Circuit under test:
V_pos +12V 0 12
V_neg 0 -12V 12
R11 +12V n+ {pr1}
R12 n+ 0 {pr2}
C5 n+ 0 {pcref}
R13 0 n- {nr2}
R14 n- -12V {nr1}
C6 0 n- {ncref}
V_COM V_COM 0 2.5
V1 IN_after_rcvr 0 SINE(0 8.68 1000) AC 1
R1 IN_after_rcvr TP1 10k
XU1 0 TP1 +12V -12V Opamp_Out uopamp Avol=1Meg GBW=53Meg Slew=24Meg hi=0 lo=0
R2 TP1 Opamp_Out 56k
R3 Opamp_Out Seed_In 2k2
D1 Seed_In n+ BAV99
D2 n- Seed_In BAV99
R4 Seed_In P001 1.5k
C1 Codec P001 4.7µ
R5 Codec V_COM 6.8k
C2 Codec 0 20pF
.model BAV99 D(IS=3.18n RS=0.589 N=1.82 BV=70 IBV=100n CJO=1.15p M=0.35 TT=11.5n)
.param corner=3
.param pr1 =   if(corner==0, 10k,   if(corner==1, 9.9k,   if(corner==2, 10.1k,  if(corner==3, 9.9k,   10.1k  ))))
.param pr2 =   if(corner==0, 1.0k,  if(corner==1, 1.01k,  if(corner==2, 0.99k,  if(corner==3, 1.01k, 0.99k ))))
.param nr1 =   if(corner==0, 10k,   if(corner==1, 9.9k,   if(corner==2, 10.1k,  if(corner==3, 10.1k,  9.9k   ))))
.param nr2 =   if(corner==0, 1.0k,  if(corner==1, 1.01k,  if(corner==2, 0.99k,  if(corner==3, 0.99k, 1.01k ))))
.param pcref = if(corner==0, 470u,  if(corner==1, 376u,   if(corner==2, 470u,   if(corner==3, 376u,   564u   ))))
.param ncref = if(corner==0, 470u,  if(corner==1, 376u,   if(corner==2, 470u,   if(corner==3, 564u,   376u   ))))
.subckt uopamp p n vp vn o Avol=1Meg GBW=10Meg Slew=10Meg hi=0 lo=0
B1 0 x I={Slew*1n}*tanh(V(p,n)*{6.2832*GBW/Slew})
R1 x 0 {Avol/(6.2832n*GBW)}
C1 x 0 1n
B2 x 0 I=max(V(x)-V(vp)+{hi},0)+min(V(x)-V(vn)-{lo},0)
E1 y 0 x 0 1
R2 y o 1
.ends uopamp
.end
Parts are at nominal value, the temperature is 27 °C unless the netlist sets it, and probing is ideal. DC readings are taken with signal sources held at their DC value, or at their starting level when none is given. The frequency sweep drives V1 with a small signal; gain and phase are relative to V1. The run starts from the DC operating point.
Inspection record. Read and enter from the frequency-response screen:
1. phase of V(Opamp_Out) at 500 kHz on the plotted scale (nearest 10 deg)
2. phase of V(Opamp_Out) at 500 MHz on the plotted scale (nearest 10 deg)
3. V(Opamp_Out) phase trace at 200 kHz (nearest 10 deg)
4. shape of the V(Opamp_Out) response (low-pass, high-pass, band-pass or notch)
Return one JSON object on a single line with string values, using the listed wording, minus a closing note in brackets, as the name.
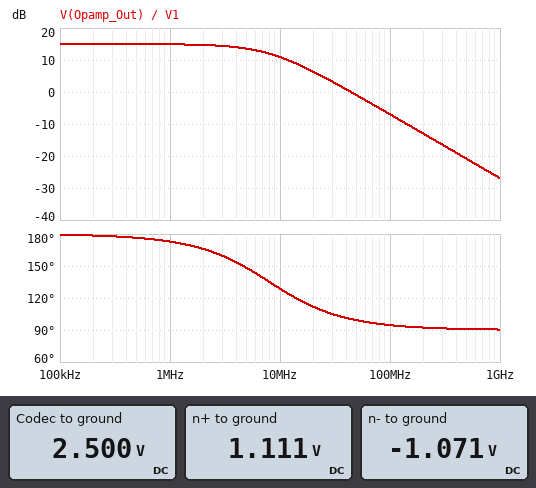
{"phase of V(Opamp_Out) at 500 kHz on the plotted scale": "180 deg", "phase of V(Opamp_Out) at 500 MHz on the plotted scale": "90 deg", "V(Opamp_Out) phase trace at 200 kHz": "180 deg", "shape of the V(Opamp_Out) response": "low-pass"}
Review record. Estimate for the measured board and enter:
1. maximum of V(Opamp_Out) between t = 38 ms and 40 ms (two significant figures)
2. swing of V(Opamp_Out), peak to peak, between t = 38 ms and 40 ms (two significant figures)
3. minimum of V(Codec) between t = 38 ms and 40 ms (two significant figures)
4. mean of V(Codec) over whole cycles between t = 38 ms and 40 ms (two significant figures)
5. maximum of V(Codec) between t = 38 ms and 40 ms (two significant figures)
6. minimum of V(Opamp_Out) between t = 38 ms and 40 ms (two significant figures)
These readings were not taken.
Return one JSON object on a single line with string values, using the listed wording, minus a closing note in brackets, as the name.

{"maximum of V(Opamp_Out) between t = 38 ms and 40 ms": "12 V", "swing of V(Opamp_Out), peak to peak, between t = 38 ms and 40 ms": "24 V", "minimum of V(Codec) between t = 38 ms and 40 ms": "940 mV", "mean of V(Codec) over whole cycles between t = 38 ms and 40 ms": "2.5 V", "maximum of V(Codec) between t = 38 ms and 40 ms": "4.1 V", "minimum of V(Opamp_Out) between t = 38 ms and 40 ms": "-12 V"}
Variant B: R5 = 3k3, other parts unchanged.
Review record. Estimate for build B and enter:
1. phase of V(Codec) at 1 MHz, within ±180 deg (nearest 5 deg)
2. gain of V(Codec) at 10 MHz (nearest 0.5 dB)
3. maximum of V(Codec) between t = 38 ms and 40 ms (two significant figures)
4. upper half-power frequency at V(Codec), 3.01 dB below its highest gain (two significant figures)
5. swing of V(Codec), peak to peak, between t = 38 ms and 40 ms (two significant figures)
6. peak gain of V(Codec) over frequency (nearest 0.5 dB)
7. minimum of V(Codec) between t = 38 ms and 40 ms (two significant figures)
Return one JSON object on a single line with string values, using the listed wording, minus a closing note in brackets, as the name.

{"phase of V(Codec) at 1 MHz, within ±180 deg": "160 deg", "gain of V(Codec) at 10 MHz": "-3.5 dB", "maximum of V(Codec) between t = 38 ms and 40 ms": "3.8 V", "upper half-power frequency at V(Codec), 3.01 dB below its highest gain": "3.6 MHz", "swing of V(Codec), peak to peak, between t = 38 ms and 40 ms": "2.7 V", "peak gain of V(Codec) over frequency": "8.5 dB", "minimum of V(Codec) between t = 38 ms and 40 ms": "1.2 V"}
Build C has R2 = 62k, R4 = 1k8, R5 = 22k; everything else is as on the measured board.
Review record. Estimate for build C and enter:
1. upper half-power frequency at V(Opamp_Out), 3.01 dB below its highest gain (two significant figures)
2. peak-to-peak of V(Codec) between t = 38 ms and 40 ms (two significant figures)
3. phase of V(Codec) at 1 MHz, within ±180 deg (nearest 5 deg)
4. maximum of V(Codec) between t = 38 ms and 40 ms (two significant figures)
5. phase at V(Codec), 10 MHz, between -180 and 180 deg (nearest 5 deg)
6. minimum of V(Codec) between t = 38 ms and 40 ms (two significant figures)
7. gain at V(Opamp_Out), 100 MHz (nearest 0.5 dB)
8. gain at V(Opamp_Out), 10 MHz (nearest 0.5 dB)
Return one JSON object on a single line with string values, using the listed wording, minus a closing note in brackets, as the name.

{"upper half-power frequency at V(Opamp_Out), 3.01 dB below its highest gain": "7.4 MHz", "peak-to-peak of V(Codec) between t = 38 ms and 40 ms": "3.6 V", "phase of V(Codec) at 1 MHz, within ±180 deg": "150 deg", "maximum of V(Codec) between t = 38 ms and 40 ms": "4.3 V", "phase at V(Codec), 10 MHz, between -180 and 180 deg": "45 deg", "minimum of V(Codec) between t = 38 ms and 40 ms": "750 mV", "gain at V(Opamp_Out), 100 MHz": "-7.0 dB", "gain at V(Opamp_Out), 10 MHz": "11.5 dB"}
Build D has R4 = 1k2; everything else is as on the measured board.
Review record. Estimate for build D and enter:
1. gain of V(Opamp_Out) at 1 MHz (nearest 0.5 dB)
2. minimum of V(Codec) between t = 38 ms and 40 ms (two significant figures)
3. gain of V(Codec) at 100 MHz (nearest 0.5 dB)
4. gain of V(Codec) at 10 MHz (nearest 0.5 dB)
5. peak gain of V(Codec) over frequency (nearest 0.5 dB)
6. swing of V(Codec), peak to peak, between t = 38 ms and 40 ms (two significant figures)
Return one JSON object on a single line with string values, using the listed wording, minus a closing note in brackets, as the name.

{"gain of V(Opamp_Out) at 1 MHz": "15.0 dB", "minimum of V(Codec) between t = 38 ms and 40 ms": "880 mV", "gain of V(Codec) at 100 MHz": "-42.0 dB", "gain of V(Codec) at 10 MHz": "-2.5 dB", "peak gain of V(Codec) over frequency": "11.5 dB", "swing of V(Codec), peak to peak, between t = 38 ms and 40 ms": "3.3 V"}
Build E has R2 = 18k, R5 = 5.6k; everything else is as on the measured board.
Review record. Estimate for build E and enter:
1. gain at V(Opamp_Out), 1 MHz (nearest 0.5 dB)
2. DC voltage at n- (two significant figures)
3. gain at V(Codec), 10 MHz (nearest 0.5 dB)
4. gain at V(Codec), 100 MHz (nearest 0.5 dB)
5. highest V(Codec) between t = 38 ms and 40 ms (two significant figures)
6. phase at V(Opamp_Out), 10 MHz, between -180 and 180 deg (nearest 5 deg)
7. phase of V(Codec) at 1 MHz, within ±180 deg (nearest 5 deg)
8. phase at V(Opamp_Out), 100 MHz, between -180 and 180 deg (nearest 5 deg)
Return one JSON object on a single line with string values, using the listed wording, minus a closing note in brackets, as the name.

{"gain at V(Opamp_Out), 1 MHz": "5.0 dB", "DC voltage at n-": "-1.1 V", "gain at V(Codec), 10 MHz": "-10.0 dB", "gain at V(Codec), 100 MHz": "-46.0 dB", "highest V(Codec) between t = 38 ms and 40 ms": "4.0 V", "phase at V(Opamp_Out), 10 MHz, between -180 and 180 deg": "150 deg", "phase of V(Codec) at 1 MHz, within ±180 deg": "160 deg", "phase at V(Opamp_Out), 100 MHz, between -180 and 180 deg": "100 deg"}
